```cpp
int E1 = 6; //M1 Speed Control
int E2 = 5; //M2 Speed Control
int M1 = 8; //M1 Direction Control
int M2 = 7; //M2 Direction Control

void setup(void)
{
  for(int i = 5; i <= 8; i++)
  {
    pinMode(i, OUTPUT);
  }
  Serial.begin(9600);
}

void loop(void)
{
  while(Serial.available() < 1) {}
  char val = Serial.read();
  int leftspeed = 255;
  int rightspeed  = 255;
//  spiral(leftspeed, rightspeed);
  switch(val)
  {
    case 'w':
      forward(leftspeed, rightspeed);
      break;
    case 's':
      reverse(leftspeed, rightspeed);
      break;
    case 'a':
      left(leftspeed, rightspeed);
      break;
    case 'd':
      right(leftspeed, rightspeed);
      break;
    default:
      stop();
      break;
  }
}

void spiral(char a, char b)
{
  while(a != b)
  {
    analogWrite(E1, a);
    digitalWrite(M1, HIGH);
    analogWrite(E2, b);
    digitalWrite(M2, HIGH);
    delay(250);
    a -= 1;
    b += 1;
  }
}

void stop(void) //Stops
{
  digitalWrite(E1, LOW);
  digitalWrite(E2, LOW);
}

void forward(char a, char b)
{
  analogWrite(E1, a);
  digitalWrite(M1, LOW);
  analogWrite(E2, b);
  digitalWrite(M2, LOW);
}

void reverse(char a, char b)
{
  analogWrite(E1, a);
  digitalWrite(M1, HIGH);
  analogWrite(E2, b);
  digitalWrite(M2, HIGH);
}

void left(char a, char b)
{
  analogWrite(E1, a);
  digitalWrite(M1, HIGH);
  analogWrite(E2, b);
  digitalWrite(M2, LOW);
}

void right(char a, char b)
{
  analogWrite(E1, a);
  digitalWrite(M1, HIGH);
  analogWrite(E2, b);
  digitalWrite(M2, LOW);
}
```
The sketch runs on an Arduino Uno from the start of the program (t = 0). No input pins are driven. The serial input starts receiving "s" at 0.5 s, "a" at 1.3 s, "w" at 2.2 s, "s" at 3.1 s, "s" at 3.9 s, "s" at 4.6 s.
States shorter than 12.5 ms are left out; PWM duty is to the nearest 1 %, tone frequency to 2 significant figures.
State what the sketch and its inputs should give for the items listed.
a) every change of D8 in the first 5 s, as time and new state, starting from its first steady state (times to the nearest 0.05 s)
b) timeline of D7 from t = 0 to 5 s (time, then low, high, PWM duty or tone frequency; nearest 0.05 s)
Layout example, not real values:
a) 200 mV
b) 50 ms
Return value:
a) 0 s low; 0.5 s high; 2.2 s low; 3.1 s high
b) 0 s low; 0.5 s high; 1.3 s low; 3.1 s high
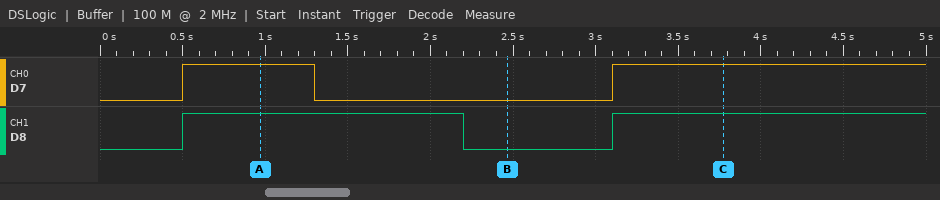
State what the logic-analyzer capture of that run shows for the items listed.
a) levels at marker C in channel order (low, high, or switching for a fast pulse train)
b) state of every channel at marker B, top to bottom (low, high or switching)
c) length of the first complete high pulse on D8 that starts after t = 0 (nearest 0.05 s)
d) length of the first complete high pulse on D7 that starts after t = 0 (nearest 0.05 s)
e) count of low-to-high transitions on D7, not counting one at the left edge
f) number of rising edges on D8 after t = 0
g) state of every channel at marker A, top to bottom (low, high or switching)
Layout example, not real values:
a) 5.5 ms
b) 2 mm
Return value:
a) D7 high, D8 high
b) D7 low, D8 low
c) 1.70 s
d) 0.80 s
e) 2
f) 2
g) D7 high, D8 high
